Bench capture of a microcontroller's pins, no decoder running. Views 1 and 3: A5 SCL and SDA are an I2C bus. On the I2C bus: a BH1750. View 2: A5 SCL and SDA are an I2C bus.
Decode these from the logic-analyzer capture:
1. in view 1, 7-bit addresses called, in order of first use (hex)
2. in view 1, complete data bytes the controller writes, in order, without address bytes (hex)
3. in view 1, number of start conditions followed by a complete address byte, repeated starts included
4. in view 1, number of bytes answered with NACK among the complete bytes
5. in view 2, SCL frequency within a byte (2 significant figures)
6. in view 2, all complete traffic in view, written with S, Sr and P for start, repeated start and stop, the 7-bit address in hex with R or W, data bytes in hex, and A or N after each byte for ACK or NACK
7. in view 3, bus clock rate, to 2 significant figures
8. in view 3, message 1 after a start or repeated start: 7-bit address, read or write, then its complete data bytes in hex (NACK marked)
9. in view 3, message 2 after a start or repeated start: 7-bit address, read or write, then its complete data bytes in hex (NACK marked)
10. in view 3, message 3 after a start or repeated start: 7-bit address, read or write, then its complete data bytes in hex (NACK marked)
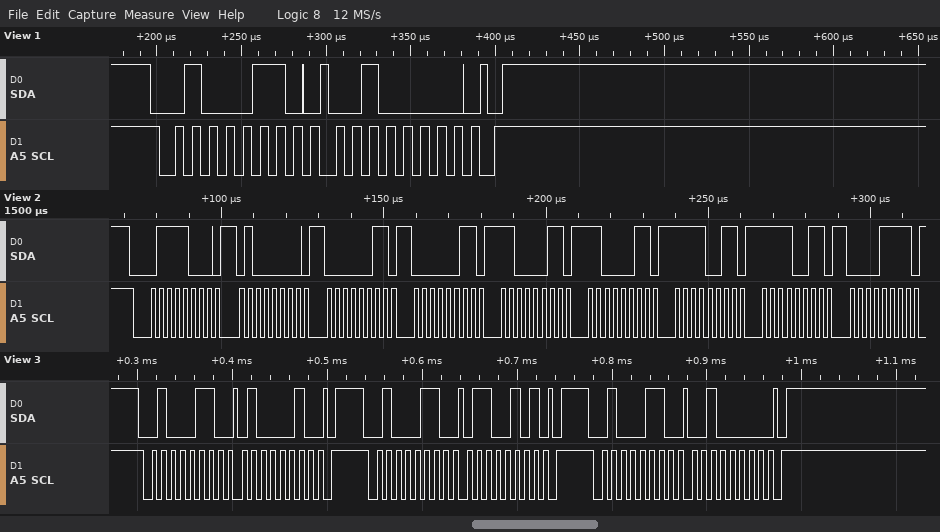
0x23
20
1
0
400 kHz
S 3CW A 40 A 03 A 03 A C3 A C3 A F3 A F3 A 0F A
100 kHz
0x23 write: 42
0x23 write: 65
0x23 write: 20
